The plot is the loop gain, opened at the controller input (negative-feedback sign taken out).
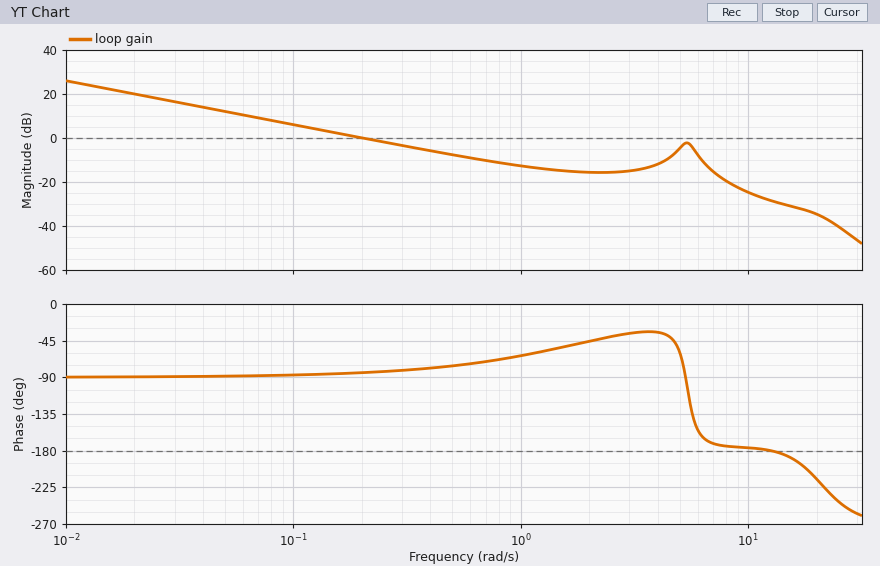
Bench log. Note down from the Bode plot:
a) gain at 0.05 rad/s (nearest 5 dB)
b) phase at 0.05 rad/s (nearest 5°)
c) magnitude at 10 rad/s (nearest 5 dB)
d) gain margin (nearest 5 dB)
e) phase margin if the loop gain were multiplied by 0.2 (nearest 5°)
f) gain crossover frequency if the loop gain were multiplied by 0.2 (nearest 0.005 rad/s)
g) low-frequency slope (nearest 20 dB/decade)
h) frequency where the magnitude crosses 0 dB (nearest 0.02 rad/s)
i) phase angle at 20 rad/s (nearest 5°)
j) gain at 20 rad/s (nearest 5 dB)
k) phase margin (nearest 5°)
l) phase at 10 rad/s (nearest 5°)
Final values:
10 dB
-90°
-25 dB
30 dB
90°
0.040 rad/s
-20 dB/decade
0.20 rad/s
-215°
-35 dB
95°
-175°
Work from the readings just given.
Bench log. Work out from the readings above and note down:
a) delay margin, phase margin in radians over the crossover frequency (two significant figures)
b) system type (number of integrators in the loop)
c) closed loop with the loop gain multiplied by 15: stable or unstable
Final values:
8.3 s
1
stable
